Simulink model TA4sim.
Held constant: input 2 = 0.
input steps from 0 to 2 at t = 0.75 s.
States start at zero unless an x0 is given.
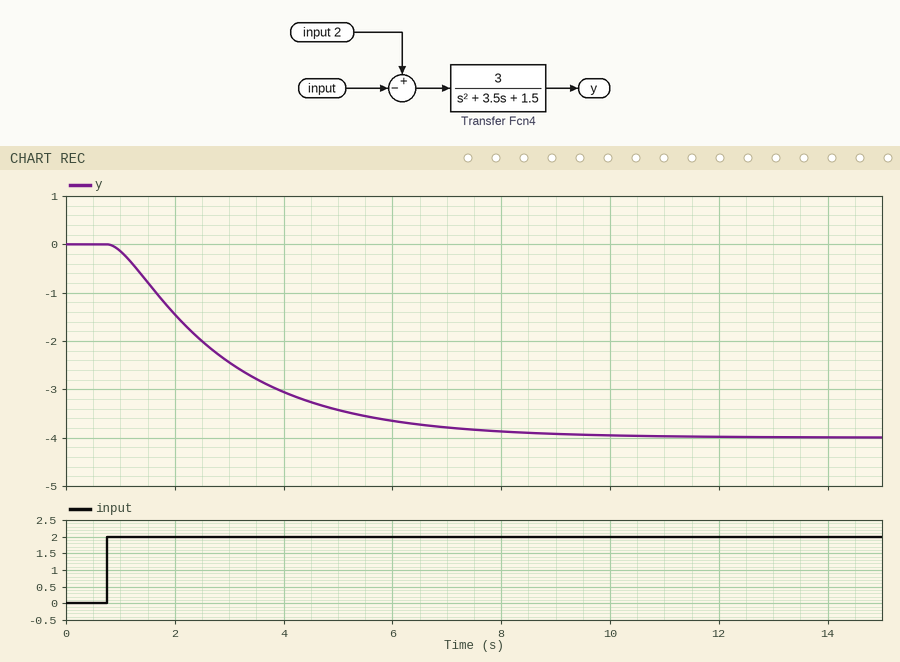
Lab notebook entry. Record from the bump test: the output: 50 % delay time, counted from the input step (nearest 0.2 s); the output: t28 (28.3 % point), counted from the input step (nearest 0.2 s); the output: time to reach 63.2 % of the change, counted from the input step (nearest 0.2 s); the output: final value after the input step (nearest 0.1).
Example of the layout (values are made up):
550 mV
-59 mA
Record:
1.8 s
1.0 s
2.4 s
-4.0
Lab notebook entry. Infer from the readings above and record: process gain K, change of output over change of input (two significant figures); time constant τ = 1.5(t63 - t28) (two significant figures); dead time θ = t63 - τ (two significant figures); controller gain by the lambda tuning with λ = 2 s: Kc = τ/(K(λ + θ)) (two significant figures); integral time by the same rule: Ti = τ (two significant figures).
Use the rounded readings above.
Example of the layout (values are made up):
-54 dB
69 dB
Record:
-2.0
2.1 s
0.30 s
-0.46
2.1 s
